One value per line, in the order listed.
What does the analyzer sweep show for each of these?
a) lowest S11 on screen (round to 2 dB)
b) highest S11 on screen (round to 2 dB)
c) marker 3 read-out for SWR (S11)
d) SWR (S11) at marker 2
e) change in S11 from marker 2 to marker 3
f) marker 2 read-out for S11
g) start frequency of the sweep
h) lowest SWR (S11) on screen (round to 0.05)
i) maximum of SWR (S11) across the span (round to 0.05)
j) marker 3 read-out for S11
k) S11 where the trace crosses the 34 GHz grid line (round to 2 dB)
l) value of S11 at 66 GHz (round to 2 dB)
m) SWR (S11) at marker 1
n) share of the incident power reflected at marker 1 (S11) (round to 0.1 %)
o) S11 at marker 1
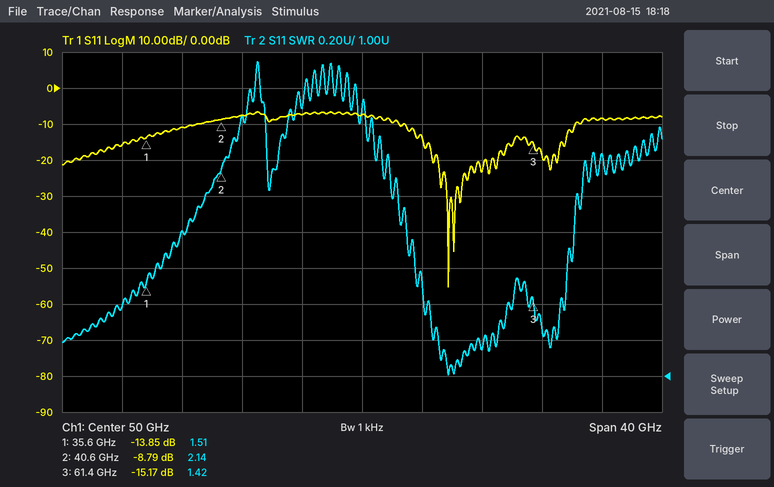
-56 dB
-6 dB
1.42
2.14
-6.38 dB
-8.79 dB
30 GHz
1.00
2.75
-15.17 dB
-16 dB
-8 dB
1.51
4.1 %
-13.85 dB
